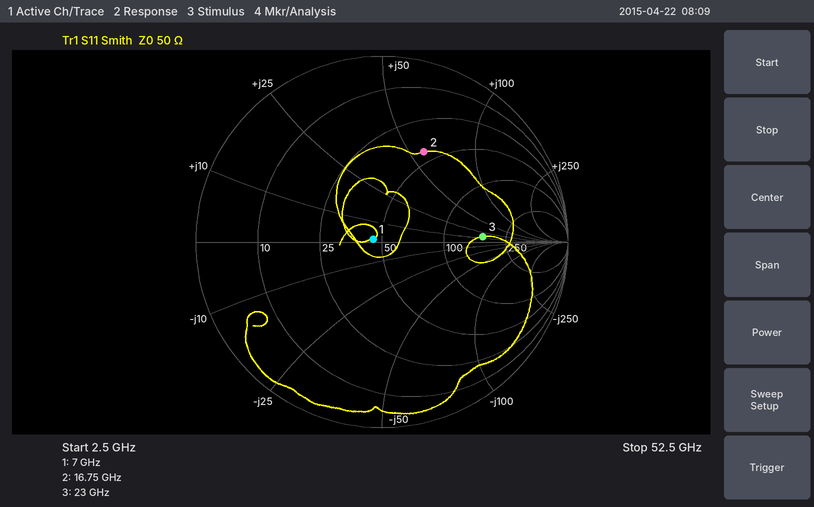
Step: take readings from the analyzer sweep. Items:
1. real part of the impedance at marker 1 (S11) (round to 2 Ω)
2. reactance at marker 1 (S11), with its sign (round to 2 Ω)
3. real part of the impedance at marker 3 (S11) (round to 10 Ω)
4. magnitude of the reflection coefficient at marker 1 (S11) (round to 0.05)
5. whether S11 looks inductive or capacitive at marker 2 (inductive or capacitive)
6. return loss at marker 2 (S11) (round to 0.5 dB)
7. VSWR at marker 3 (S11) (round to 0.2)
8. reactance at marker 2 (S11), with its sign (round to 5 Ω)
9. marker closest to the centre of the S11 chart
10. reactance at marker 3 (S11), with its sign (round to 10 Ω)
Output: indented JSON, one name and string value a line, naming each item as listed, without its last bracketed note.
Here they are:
{
  "real part of the impedance at marker 1 (S11)": "46 Ω",
  "reactance at marker 1 (S11), with its sign": "+2 Ω",
  "real part of the impedance at marker 3 (S11)": "170 Ω",
  "magnitude of the reflection coefficient at marker 1 (S11)": "0.05",
  "whether S11 looks inductive or capacitive at marker 2": "inductive",
  "return loss at marker 2 (S11)": "5.5 dB",
  "VSWR at marker 3 (S11)": "3.4",
  "reactance at marker 2 (S11), with its sign": "+60 Ω",
  "marker closest to the centre of the S11 chart": "marker 1",
  "reactance at marker 3 (S11), with its sign": "+10 Ω"
}
